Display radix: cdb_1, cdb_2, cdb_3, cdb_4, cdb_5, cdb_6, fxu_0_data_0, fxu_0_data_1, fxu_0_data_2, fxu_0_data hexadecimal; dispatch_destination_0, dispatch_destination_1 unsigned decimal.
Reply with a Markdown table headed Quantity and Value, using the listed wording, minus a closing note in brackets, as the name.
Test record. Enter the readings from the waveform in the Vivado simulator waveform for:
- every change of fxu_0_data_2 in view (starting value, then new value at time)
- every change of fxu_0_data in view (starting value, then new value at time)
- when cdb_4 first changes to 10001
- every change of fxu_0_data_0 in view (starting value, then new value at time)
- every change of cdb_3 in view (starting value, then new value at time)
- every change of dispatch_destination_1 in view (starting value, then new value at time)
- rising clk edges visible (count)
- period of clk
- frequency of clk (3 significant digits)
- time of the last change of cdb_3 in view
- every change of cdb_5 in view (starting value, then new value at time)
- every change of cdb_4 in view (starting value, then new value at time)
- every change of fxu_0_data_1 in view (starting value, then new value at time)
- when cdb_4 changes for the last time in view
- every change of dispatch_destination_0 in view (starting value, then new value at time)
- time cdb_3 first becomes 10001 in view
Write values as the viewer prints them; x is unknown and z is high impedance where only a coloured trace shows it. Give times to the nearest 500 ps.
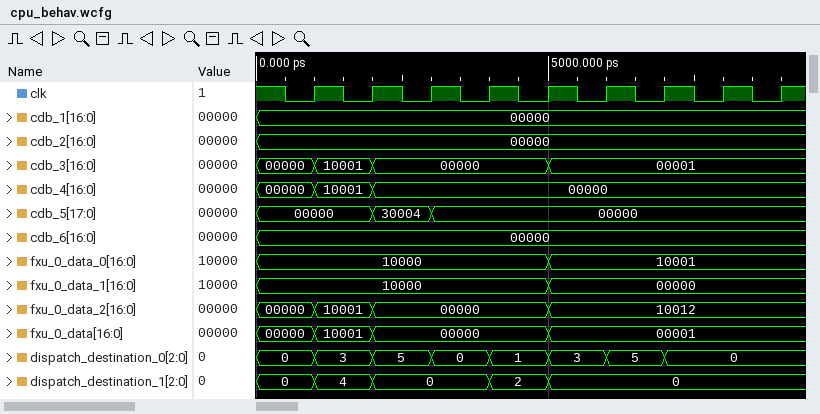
| Quantity | Value |
|---|---|
| every change of fxu_0_data_2 in view | 00000, 10001 at 1000 ps, 00000 at 2000 ps, 10012 at 5000 ps |
| every change of fxu_0_data in view | 00000, 10001 at 1000 ps, 00000 at 2000 ps, 00001 at 5000 ps |
| when cdb_4 first changes to 10001 | 1000 ps |
| every change of fxu_0_data_0 in view | 10000, 10001 at 5000 ps |
| every change of cdb_3 in view | 00000, 10001 at 1000 ps, 00000 at 2000 ps, 00001 at 5000 ps |
| every change of dispatch_destination_1 in view | 0, 4 at 1000 ps, 0 at 2000 ps, 2 at 4000 ps, 0 at 5000 ps |
| rising clk edges visible | 9 |
| period of clk | 1000 ps |
| frequency of clk | 1.00 GHz |
| time of the last change of cdb_3 in view | 5000 ps |
| every change of cdb_5 in view | 00000, 30004 at 2000 ps, 00000 at 3000 ps |
| every change of cdb_4 in view | 00000, 10001 at 1000 ps, 00000 at 2000 ps |
| every change of fxu_0_data_1 in view | 10000, 00000 at 5000 ps |
| when cdb_4 changes for the last time in view | 2000 ps |
| every change of dispatch_destination_0 in view | 0, 3 at 1000 ps, 5 at 2000 ps, 0 at 3000 ps, 1 at 4000 ps, 3 at 5000 ps, 5 at 6000 ps, 0 at 7000 ps |
| time cdb_3 first becomes 10001 in view | 1000 ps |
